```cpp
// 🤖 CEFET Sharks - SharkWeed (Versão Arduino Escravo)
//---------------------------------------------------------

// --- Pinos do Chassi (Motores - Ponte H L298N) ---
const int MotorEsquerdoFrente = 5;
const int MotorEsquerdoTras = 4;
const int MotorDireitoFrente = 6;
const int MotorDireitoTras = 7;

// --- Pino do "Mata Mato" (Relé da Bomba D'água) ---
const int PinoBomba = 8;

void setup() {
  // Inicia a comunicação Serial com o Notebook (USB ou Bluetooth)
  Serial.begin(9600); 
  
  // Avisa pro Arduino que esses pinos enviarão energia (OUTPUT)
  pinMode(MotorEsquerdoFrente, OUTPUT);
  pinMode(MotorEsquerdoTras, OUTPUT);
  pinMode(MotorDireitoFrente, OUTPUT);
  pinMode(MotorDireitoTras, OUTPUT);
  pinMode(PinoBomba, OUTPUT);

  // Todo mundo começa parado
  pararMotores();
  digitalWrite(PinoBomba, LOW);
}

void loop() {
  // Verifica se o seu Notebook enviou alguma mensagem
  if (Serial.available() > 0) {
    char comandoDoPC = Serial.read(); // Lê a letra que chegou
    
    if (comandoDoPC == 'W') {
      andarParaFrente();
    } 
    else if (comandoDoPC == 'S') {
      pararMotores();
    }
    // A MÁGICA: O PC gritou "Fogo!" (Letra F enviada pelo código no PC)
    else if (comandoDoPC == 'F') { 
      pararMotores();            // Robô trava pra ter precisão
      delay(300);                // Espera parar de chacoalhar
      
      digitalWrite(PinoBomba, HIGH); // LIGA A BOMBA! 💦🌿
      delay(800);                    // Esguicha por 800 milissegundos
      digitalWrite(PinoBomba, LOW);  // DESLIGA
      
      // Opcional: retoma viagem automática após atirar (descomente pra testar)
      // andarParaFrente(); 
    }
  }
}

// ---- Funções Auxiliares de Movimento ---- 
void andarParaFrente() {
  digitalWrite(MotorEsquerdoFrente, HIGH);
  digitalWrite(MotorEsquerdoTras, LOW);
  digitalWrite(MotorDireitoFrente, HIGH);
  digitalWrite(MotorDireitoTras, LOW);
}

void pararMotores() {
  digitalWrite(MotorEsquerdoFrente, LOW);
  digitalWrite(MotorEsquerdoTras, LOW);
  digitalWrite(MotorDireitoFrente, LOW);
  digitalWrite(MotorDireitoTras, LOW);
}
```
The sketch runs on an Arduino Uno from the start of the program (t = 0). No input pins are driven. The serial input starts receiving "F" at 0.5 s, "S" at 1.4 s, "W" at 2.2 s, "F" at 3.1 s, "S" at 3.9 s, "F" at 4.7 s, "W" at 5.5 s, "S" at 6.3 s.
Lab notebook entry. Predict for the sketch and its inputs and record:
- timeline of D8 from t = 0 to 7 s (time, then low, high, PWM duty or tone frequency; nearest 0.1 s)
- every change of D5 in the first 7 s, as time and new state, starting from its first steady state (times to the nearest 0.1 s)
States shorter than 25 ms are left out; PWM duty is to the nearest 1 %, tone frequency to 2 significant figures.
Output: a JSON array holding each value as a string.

["0 s low; 0.8 s high; 1.6 s low; 3.4 s high; 4.2 s low; 5 s high; 5.8 s low", "0 s low; 2.2 s high; 3.1 s low; 5.8 s high; 6.3 s low"]
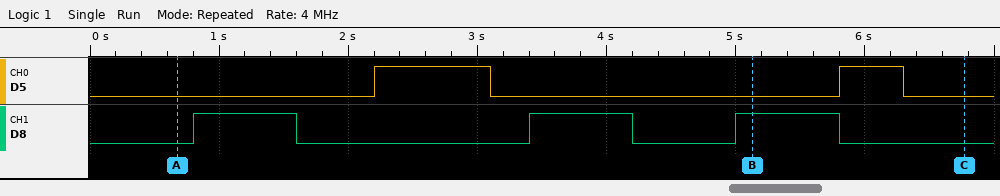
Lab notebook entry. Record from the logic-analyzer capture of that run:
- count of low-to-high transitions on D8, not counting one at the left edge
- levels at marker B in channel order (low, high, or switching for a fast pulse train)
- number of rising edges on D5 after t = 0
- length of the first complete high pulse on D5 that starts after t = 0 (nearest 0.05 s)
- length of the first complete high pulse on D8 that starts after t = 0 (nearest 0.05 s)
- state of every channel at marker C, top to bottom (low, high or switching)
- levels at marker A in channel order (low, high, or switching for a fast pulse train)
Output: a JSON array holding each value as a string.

["3", "D5 low, D8 high", "2", "0.90 s", "0.80 s", "D5 low, D8 low", "D5 low, D8 low"]
